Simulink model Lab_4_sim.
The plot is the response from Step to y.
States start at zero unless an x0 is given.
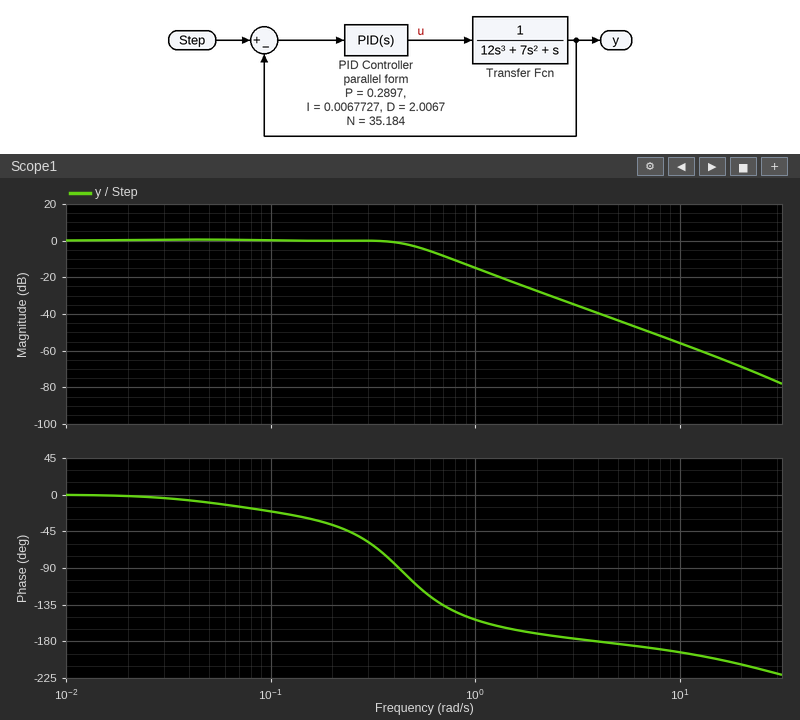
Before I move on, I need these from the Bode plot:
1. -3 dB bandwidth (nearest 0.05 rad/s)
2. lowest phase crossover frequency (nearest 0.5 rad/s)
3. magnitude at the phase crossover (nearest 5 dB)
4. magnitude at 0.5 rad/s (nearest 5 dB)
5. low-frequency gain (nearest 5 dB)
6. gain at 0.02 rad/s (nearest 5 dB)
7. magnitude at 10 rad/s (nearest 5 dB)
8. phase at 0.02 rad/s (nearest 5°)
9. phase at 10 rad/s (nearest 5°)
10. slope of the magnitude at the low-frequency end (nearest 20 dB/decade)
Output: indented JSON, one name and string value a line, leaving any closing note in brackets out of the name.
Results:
{
  "-3 dB bandwidth": "0.50 rad/s",
  "lowest phase crossover frequency": "4.0 rad/s",
  "magnitude at the phase crossover": "-40 dB",
  "magnitude at 0.5 rad/s": "-5 dB",
  "low-frequency gain": "0 dB",
  "gain at 0.02 rad/s": "0 dB",
  "magnitude at 10 rad/s": "-55 dB",
  "phase at 0.02 rad/s": "0°",
  "phase at 10 rad/s": "-195°",
  "slope of the magnitude at the low-frequency end": "0 dB/decade"
}
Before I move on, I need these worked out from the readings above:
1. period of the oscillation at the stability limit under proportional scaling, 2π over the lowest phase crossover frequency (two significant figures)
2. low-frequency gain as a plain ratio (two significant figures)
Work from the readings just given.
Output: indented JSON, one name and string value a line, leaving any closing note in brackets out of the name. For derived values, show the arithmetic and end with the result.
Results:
{
  "period of the oscillation at the stability limit under proportional scaling, 2π over the lowest phase crossover frequency": "2π / 4 = 1.6 s",
  "low-frequency gain as a plain ratio": "10^(0 / 20) = 1.0"
}
